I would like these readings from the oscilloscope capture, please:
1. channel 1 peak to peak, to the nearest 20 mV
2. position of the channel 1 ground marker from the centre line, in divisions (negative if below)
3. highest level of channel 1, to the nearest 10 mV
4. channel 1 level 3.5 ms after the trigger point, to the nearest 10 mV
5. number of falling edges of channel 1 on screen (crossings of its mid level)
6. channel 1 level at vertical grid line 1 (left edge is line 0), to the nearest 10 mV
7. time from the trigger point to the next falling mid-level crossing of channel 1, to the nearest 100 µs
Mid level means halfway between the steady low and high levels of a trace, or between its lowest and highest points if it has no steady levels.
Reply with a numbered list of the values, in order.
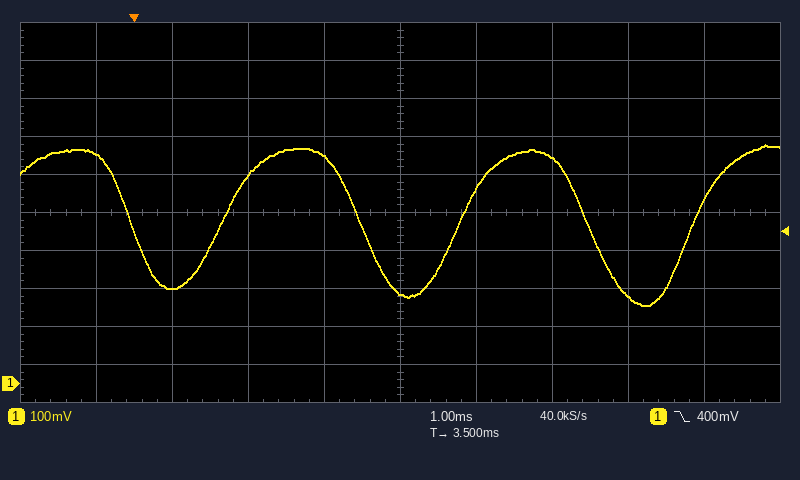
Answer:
1. 420 mV
2. -4.5 div
3. 630 mV
4. 240 mV
5. 3
6. 600 mV
7. 3.0 ms
